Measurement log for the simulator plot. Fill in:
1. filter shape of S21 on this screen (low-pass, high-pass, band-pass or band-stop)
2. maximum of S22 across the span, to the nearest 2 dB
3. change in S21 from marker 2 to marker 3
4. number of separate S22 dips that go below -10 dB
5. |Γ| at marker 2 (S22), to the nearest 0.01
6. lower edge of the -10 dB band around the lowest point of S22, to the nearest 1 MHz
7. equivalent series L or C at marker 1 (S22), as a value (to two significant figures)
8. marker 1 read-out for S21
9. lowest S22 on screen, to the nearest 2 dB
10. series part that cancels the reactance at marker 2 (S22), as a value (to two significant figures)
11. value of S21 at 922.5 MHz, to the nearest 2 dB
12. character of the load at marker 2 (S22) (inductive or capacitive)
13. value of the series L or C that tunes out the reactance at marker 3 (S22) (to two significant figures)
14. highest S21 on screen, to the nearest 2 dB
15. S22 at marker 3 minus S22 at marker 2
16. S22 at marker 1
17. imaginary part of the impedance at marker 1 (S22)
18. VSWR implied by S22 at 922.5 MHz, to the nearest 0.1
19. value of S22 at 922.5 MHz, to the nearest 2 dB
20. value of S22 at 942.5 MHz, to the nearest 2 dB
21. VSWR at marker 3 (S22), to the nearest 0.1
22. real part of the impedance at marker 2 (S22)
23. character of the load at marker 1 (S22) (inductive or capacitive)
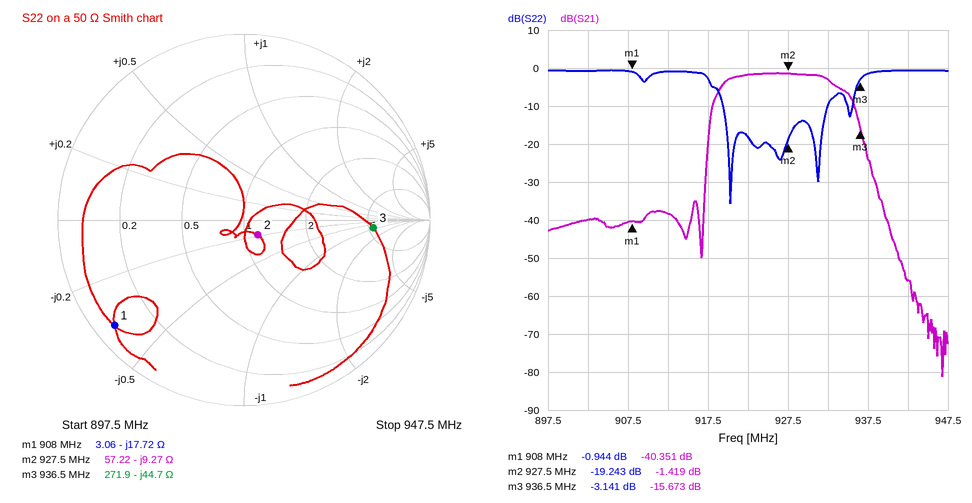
band-pass
0 dB
-14.254 dB
4
0.11
919 MHz
9.9 pF
-40.351 dB
-36 dB
1.6 nH
-2 dB
capacitive
7.6 nH
-2 dB
16.102 dB
-0.944 dB
-17.72 Ω
1.3
-18 dB
0 dB
5.6
57.22 Ω
capacitive
